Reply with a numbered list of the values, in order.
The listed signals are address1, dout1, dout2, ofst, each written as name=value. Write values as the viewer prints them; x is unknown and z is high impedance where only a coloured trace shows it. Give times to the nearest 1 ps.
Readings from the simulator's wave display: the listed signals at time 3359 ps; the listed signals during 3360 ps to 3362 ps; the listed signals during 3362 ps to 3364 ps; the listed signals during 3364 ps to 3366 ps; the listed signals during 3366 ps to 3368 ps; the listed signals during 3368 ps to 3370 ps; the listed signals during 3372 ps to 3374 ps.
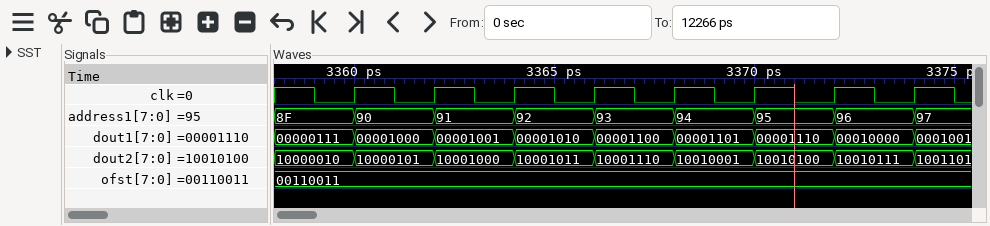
1. address1=8F, dout1=00000111, dout2=10000010, ofst=00110011
2. address1=90, dout1=00001000, dout2=10000101, ofst=00110011
3. address1=91, dout1=00001001, dout2=10001000, ofst=00110011
4. address1=92, dout1=00001010, dout2=10001011, ofst=00110011
5. address1=93, dout1=00001100, dout2=10001110, ofst=00110011
6. address1=94, dout1=00001101, dout2=10010001, ofst=00110011
7. address1=96, dout1=00010000, dout2=10010111, ofst=00110011
